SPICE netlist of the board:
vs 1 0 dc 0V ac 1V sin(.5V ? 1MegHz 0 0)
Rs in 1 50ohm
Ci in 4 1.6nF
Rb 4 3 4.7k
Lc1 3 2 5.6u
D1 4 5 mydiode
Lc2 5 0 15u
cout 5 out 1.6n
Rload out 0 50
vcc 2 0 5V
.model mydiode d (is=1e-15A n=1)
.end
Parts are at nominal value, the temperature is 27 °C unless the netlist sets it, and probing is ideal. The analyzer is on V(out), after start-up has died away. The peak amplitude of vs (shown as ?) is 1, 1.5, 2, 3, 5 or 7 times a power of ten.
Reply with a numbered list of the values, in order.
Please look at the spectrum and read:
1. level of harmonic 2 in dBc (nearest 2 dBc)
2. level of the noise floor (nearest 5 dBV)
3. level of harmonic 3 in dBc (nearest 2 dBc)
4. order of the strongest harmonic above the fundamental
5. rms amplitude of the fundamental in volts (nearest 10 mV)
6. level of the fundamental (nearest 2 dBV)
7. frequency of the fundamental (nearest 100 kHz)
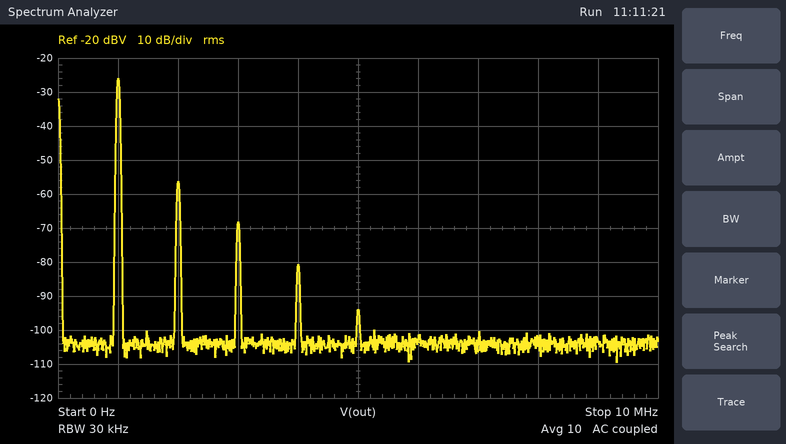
1. -30 dBc
2. -105 dBV
3. -42 dBc
4. 2
5. 50 mV
6. -26 dBV
7. 1.0 MHz
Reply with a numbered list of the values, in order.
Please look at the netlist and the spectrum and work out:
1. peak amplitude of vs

1. 200 mV
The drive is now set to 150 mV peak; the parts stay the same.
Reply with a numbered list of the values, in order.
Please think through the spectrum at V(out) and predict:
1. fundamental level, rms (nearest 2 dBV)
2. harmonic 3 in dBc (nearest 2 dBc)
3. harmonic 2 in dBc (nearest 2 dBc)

1. -28 dBV
2. -48 dBc
3. -34 dBc
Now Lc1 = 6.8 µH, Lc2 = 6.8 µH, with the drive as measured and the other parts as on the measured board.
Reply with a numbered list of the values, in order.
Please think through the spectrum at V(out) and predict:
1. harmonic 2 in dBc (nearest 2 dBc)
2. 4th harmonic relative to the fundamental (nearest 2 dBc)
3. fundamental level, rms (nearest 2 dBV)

1. -6 dBc
2. -34 dBc
3. -32 dBV
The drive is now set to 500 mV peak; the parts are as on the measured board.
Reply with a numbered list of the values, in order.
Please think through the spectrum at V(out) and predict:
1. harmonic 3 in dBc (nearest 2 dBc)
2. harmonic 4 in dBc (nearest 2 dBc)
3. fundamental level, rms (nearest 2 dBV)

1. -28 dBc
2. -30 dBc
3. -20 dBV
